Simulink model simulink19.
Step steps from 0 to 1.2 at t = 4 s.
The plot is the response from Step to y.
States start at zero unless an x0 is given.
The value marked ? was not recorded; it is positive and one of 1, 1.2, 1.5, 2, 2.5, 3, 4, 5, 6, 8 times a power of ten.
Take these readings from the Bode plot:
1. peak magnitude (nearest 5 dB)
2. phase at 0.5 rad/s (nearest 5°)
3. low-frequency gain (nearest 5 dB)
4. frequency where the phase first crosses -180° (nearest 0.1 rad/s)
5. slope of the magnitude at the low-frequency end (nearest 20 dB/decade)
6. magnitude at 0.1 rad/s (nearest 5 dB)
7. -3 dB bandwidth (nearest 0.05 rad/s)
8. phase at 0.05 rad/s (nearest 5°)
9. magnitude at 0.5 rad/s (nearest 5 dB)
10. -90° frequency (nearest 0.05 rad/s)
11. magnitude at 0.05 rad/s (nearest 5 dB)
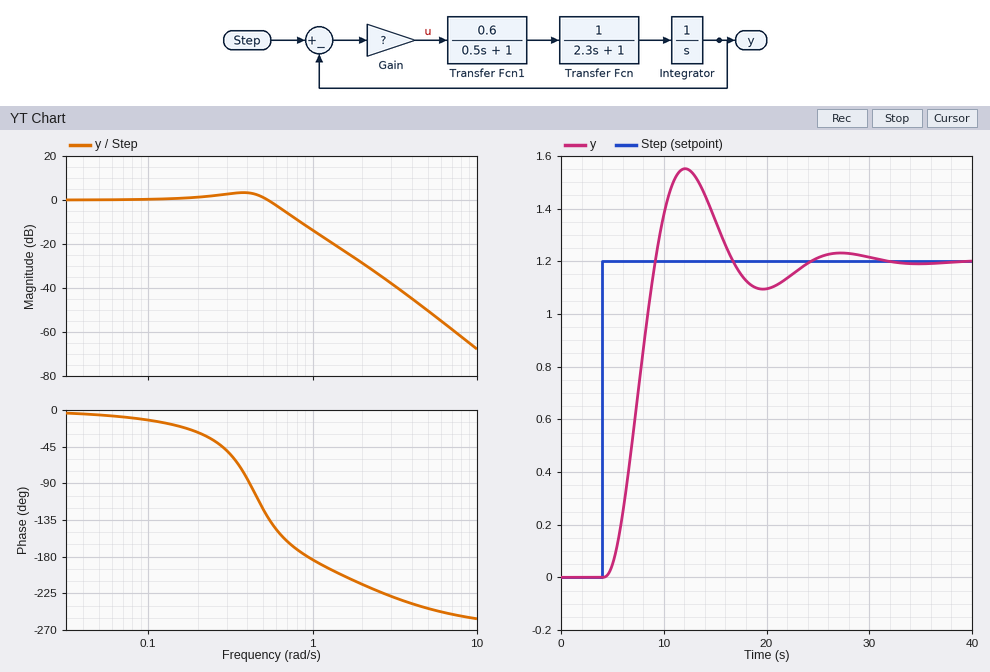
5 dB
-120°
0 dB
0.9 rad/s
0 dB/decade
0 dB
0.60 rad/s
-5°
0 dB
0.40 rad/s
0 dB
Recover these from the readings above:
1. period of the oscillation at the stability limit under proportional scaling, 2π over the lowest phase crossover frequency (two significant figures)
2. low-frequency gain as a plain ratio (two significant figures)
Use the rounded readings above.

7.0 s
1.0
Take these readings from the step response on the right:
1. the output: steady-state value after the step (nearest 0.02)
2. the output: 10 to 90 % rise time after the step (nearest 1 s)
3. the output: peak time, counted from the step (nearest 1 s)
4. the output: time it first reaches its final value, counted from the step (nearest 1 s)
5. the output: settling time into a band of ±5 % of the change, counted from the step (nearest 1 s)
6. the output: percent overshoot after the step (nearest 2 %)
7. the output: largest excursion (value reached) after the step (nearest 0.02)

1.20
3 s
8 s
5 s
18 s
30 %
1.56
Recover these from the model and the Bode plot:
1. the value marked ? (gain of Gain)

0.8
